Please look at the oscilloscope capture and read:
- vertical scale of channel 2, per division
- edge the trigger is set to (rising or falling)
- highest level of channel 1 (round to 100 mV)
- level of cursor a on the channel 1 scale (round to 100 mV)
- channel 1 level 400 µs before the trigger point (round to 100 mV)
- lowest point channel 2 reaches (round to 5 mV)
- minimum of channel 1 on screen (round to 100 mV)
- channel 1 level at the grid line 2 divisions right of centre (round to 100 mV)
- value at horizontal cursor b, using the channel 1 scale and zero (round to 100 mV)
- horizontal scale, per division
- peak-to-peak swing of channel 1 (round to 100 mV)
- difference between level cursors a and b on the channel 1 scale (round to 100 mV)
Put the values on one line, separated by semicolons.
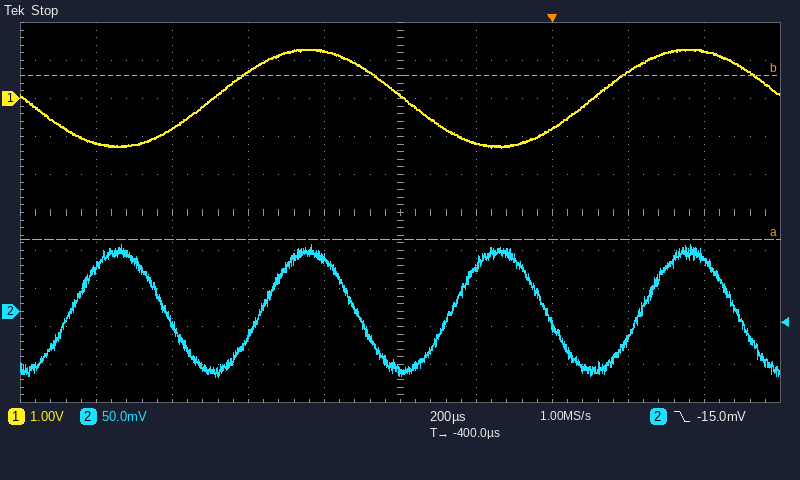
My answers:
50 mV; falling; 1.3 V; -3.7 V; 100 mV; -85 mV; -1.3 V; -800 mV; 600 mV; 200 µs; 2.6 V; 4.3 V
